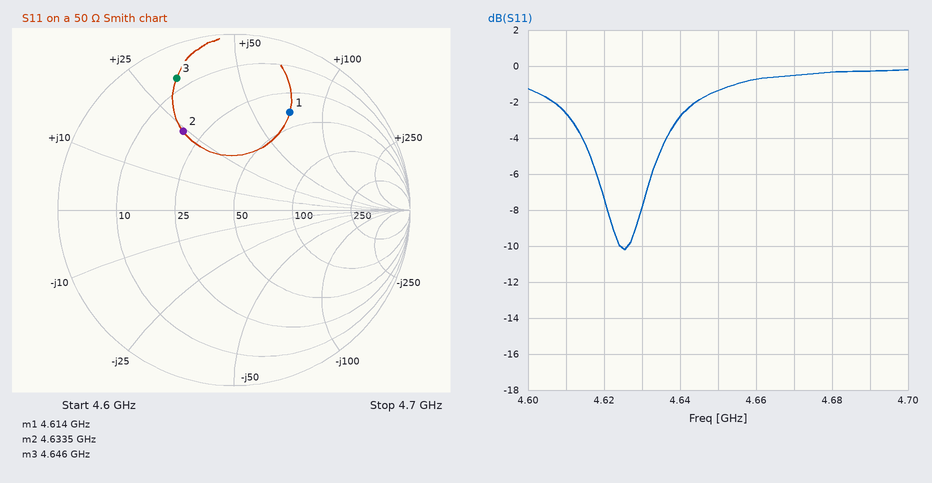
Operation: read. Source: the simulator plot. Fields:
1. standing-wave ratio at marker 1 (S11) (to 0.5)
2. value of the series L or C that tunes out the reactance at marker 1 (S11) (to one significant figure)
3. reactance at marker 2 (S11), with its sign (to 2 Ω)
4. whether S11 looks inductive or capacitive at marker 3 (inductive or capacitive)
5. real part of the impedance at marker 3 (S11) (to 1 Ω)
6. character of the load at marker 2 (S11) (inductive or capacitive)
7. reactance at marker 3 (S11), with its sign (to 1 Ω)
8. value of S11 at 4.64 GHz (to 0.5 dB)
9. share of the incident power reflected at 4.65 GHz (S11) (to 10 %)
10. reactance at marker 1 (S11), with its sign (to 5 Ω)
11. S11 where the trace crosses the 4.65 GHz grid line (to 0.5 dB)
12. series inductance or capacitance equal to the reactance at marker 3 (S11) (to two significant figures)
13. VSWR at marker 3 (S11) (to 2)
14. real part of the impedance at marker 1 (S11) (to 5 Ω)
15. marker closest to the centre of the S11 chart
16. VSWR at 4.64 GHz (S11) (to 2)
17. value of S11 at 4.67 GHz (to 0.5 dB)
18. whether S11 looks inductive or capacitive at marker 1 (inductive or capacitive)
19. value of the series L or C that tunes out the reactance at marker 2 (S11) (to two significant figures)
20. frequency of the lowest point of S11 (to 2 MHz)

4.5
500 fF
+24 Ω
inductive
7 Ω
inductive
+32 Ω
-3.0 dB
70 %
+70 Ω
-1.5 dB
1.1 nH
10
40 Ω
marker 2
6
-0.5 dB
inductive
1.4 pF
4.626 GHz
